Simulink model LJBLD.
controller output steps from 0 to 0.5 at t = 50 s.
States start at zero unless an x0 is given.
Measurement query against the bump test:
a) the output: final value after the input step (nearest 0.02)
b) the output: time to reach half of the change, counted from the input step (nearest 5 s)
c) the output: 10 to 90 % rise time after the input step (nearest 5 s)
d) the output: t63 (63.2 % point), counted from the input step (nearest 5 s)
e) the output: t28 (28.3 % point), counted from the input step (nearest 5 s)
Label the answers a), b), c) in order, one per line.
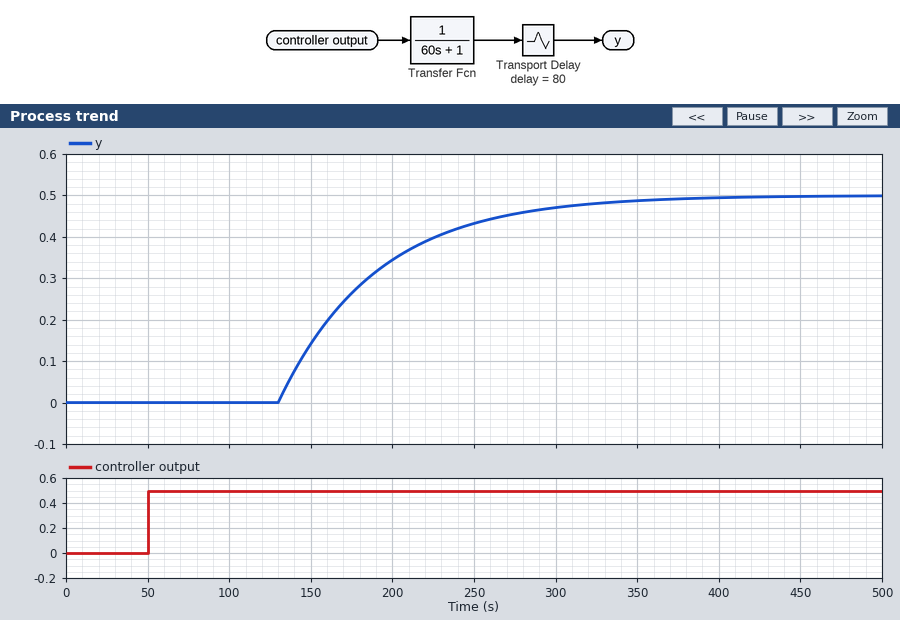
a) 0.50
b) 120 s
c) 130 s
d) 140 s
e) 100 s
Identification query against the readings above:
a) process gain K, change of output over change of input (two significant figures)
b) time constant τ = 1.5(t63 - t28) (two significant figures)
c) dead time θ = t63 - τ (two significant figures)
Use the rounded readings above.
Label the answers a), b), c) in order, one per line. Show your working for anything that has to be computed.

a) (0.5 - 0) / 0.5 = 1.0
b) 1.5 × (140 - 100) = 60 s
c) 140 - 60 = 80 s
